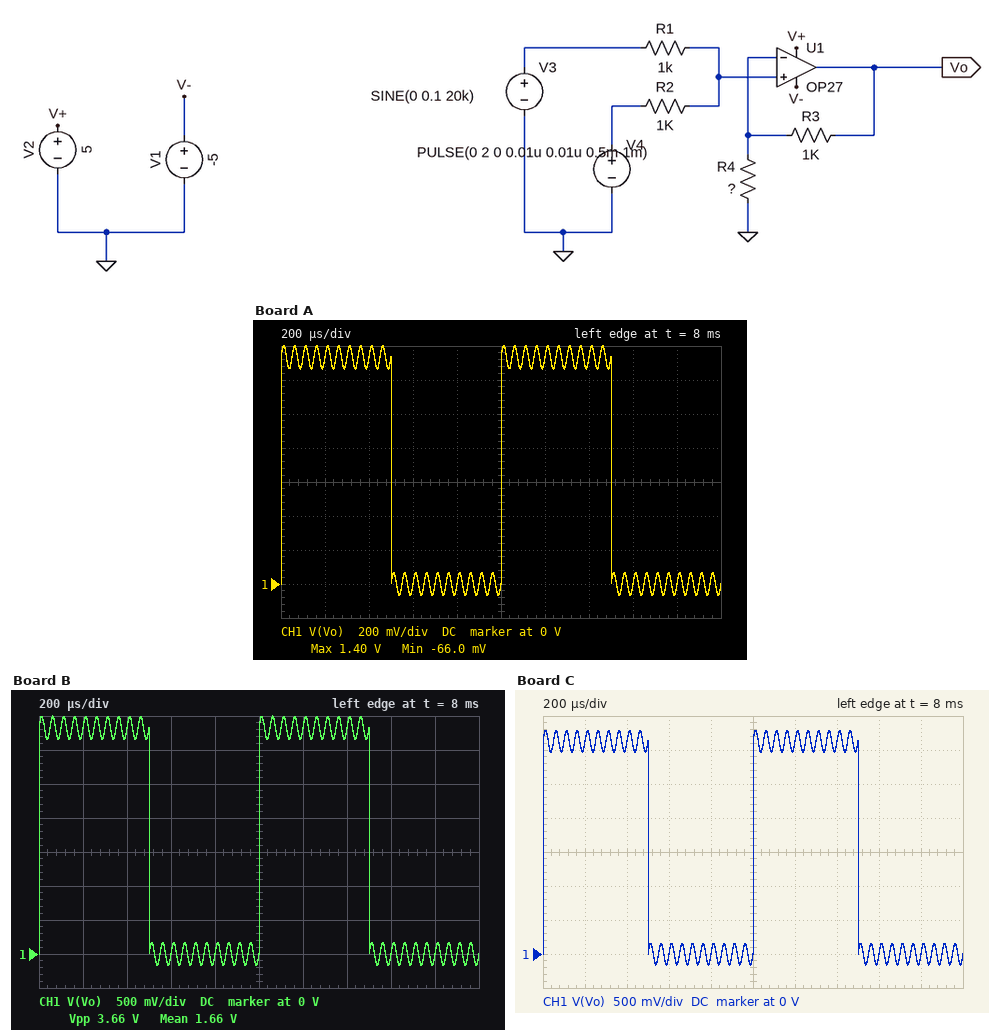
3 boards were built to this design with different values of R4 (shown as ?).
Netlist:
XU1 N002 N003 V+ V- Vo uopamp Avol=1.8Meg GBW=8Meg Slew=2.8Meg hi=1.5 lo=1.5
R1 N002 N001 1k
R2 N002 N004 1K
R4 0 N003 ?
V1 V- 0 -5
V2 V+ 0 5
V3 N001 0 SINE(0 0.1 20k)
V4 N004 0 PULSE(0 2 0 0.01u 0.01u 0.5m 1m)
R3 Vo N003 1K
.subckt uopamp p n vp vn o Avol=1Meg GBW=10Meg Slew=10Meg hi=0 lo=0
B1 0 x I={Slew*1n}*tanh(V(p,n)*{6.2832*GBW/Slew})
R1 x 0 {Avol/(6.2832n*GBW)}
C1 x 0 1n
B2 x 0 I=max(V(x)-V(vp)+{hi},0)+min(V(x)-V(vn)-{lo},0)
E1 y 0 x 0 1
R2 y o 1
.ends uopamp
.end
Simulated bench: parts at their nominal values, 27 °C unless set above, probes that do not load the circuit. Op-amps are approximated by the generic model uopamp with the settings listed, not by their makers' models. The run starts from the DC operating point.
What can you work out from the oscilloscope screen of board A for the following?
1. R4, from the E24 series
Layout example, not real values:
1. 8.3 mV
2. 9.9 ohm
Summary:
1. 3 kΩ
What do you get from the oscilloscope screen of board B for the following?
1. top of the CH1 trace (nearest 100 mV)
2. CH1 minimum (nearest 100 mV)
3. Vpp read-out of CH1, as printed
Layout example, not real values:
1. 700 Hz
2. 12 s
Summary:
1. 3.5 V
2. -200 mV
3. 3.66 V
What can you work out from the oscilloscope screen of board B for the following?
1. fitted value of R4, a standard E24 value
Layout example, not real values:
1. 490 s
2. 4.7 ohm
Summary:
1. 430 Ω
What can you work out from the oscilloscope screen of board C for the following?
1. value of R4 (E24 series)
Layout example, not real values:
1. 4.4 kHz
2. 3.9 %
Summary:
1. 470 Ω
